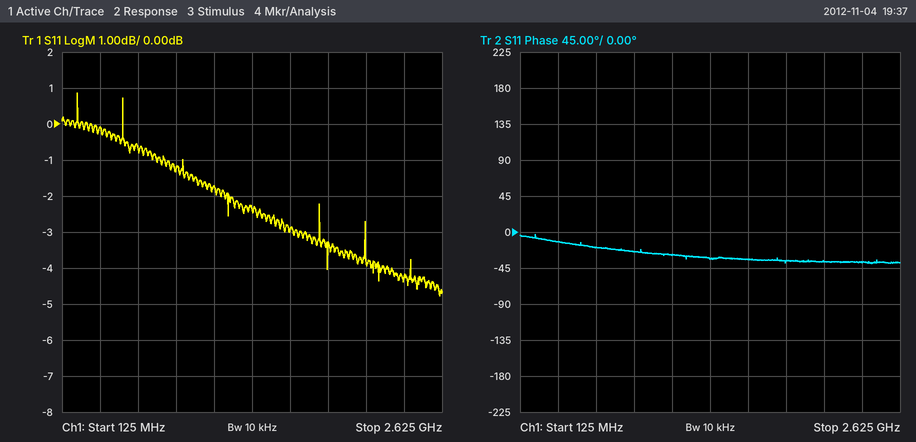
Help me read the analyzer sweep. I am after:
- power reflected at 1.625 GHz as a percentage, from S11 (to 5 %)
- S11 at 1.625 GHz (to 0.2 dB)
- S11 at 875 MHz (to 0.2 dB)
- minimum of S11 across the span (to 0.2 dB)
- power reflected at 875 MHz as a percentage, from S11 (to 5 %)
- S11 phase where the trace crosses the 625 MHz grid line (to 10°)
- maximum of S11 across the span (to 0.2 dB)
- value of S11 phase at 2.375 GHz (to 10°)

50 %
-3.0 dB
-1.2 dB
-4.8 dB
75 %
-20°
0.8 dB
-40°
